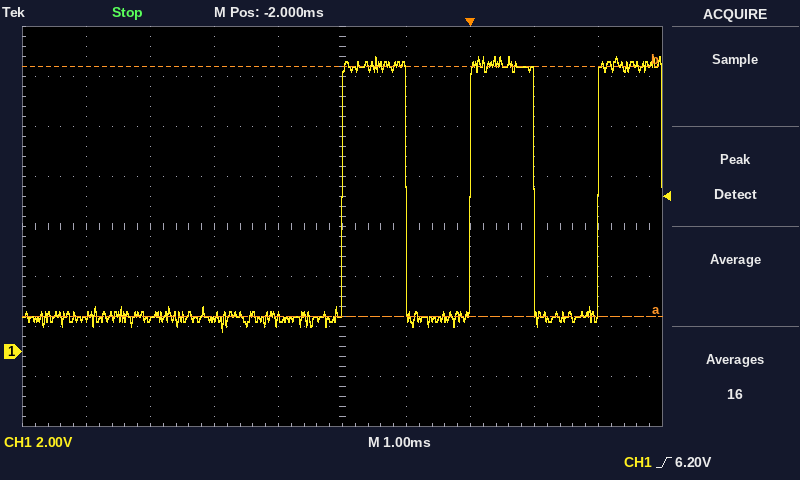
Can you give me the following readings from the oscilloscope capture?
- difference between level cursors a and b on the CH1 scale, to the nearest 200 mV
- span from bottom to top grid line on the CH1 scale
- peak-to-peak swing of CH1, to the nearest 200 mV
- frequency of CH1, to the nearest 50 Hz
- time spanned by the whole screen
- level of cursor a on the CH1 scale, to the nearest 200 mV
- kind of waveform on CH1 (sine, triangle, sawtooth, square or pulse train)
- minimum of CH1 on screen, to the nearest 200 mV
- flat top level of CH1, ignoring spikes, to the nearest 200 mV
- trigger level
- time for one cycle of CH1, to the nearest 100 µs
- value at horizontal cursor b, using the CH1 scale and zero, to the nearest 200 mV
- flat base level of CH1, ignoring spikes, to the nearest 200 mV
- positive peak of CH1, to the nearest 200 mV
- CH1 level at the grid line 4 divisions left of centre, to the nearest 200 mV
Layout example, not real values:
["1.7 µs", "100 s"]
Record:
["10.0 V", "16 V", "11.0 V", "500 Hz", "10 ms", "1.4 V", "square", "800 mV", "11.4 V", "6.20 V", "2.0 ms", "11.4 V", "1.4 V", "11.8 V", "1.4 V"]
